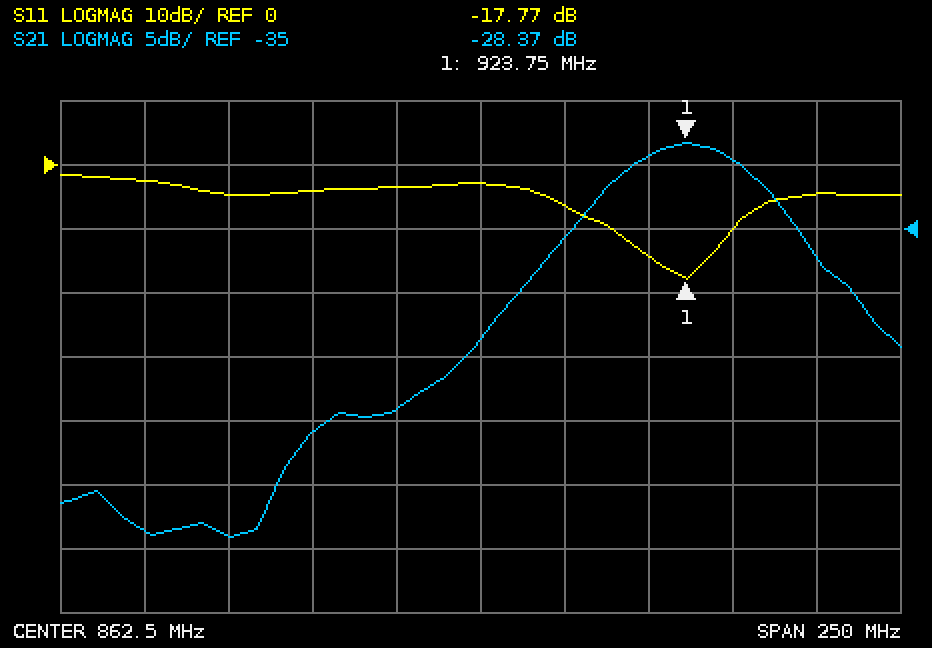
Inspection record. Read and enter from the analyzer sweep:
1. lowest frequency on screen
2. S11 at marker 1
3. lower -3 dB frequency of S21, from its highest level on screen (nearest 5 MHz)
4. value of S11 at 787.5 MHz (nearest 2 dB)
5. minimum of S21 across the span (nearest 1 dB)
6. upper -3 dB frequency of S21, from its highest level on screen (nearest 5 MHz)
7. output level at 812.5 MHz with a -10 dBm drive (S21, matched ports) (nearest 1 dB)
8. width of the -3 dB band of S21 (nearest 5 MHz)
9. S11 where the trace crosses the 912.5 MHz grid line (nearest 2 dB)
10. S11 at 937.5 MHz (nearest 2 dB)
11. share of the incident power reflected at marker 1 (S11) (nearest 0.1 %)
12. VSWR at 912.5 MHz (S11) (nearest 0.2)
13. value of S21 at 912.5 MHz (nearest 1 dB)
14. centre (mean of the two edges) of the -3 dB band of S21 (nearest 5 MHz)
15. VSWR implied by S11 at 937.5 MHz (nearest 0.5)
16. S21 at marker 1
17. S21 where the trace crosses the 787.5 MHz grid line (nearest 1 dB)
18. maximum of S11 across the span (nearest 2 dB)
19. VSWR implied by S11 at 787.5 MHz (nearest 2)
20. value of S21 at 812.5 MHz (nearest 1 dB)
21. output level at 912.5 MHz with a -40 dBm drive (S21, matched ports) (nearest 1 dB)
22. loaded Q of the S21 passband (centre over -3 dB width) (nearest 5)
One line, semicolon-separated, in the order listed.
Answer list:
737.5 MHz; -17.77 dB; 900 MHz; -4 dB; -59 dB; 945 MHz; -61 dBm; 45 MHz; -14 dB; -10 dB; 1.7 %; 1.4; -29 dB; 925 MHz; 2.0; -28.37 dB; -59 dB; -2 dB; 4; -51 dB; -69 dBm; 20
